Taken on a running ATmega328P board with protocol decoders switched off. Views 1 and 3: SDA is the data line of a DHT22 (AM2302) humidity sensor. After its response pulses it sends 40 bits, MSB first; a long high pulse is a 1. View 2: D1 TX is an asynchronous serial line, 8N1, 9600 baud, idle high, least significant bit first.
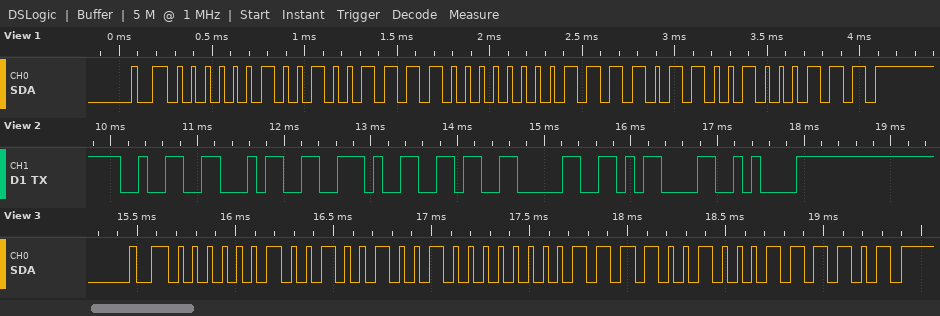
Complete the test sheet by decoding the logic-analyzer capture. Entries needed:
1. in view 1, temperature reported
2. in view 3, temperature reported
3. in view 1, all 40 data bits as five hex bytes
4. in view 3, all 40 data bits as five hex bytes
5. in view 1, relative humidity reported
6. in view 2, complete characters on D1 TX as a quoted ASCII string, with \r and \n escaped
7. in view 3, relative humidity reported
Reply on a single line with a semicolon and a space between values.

24.6 °C; 24.2 °C; 02 4F 00 F6 47; 02 49 00 F2 3D; 59.1 %; "24.60\r\n"; 58.5 %
